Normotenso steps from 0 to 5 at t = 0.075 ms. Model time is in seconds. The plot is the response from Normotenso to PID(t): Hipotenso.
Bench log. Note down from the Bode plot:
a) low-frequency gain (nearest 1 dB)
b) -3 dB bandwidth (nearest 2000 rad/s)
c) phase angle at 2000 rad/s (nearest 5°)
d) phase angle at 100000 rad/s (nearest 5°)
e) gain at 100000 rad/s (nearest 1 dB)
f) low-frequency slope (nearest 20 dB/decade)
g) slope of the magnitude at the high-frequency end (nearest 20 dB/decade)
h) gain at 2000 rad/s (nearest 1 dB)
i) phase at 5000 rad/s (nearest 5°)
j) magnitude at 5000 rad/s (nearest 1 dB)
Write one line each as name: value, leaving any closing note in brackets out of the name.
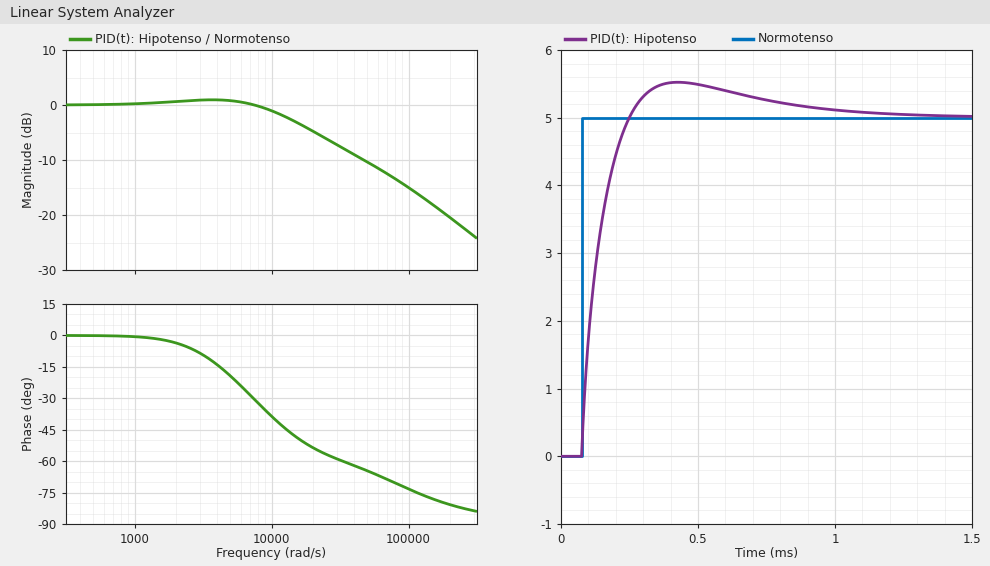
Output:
low-frequency gain: 0 dB
-3 dB bandwidth: 14000 rad/s
phase angle at 2000 rad/s: -5°
phase angle at 100000 rad/s: -75°
gain at 100000 rad/s: -15 dB
low-frequency slope: 0 dB/decade
slope of the magnitude at the high-frequency end: -20 dB/decade
gain at 2000 rad/s: 1 dB
phase at 5000 rad/s: -20°
magnitude at 5000 rad/s: 1 dB
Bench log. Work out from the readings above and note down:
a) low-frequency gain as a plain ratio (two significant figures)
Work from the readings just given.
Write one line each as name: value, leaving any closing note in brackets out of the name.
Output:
low-frequency gain as a plain ratio: 1.0
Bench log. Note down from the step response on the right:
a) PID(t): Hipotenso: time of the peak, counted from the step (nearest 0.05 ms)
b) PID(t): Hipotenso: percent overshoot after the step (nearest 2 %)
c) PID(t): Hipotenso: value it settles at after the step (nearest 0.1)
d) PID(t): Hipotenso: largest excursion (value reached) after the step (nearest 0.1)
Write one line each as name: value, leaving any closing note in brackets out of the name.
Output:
PID(t): Hipotenso: time of the peak, counted from the step: 0.35 ms
PID(t): Hipotenso: percent overshoot after the step: 10 %
PID(t): Hipotenso: value it settles at after the step: 5.0
PID(t): Hipotenso: largest excursion (value reached) after the step: 5.5
